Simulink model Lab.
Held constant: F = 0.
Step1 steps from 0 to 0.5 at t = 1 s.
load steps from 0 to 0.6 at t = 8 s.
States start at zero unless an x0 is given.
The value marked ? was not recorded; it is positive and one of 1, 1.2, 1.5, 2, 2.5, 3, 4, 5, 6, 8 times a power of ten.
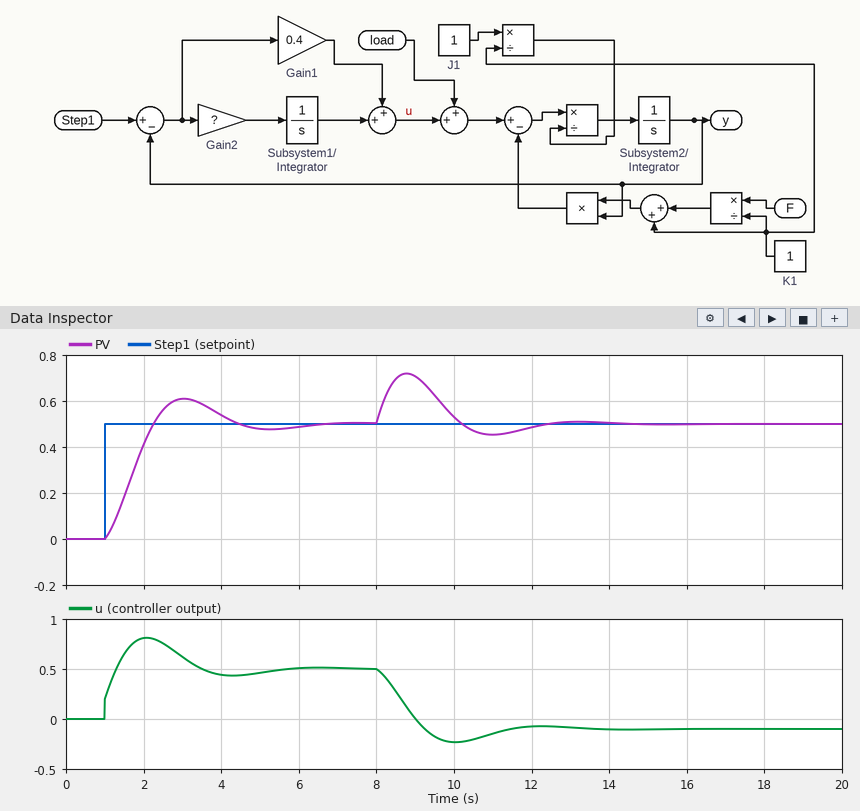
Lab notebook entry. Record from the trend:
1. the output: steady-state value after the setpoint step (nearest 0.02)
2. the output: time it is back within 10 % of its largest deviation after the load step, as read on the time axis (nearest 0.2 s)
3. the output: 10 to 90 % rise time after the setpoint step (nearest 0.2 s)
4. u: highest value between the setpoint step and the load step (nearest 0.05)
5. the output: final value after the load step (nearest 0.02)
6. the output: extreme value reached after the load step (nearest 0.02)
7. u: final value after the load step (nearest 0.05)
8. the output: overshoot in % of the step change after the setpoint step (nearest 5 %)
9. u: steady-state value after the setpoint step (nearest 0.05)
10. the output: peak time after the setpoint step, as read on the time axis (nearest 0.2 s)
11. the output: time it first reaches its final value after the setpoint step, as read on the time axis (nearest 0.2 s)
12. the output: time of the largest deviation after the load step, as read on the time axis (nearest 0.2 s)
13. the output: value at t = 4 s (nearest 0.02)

0.50
11.8 s
1.0 s
0.80
0.50
0.72
-0.10
20 %
0.50
3.0 s
2.2 s
8.8 s
0.54
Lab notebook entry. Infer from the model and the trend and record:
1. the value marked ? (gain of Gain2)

2.5
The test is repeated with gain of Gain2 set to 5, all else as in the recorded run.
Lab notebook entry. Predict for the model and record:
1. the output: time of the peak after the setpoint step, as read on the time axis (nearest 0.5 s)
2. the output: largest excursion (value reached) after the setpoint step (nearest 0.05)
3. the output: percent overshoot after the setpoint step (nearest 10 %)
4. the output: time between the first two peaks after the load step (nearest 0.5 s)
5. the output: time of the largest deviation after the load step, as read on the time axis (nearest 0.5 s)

2.5 s
0.70
40 %
3.0 s
8.5 s
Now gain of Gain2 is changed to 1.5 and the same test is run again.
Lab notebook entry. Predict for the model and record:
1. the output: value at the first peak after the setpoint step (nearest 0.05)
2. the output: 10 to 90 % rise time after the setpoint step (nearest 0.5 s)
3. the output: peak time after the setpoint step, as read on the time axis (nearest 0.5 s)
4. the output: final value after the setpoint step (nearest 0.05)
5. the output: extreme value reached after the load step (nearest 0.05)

0.55
1.5 s
4.0 s
0.50
0.75
